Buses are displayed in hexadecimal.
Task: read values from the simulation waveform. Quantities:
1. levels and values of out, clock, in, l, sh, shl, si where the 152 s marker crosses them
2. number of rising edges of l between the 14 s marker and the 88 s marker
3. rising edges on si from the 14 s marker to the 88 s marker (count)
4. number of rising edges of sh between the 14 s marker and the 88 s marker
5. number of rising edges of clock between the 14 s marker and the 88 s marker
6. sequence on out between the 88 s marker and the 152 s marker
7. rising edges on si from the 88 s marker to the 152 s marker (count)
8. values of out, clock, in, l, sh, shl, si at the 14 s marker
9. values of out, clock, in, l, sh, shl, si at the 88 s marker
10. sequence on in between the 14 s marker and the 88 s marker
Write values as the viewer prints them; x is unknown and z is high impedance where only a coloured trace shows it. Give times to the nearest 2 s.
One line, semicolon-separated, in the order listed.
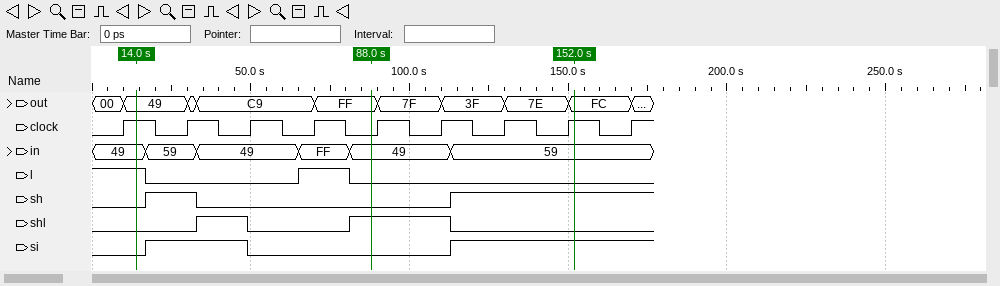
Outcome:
out=FC, clock=1, in=59, l=0, sh=1, shl=0, si=1; 1; 1; 1; 3; FF, 7F, 3F, 7E, FC; 1; out=49, clock=1, in=49, l=1, sh=0, shl=0, si=0; out=FF, clock=0, in=49, l=0, sh=0, shl=1, si=0; 49, 59, 49, FF, 49
